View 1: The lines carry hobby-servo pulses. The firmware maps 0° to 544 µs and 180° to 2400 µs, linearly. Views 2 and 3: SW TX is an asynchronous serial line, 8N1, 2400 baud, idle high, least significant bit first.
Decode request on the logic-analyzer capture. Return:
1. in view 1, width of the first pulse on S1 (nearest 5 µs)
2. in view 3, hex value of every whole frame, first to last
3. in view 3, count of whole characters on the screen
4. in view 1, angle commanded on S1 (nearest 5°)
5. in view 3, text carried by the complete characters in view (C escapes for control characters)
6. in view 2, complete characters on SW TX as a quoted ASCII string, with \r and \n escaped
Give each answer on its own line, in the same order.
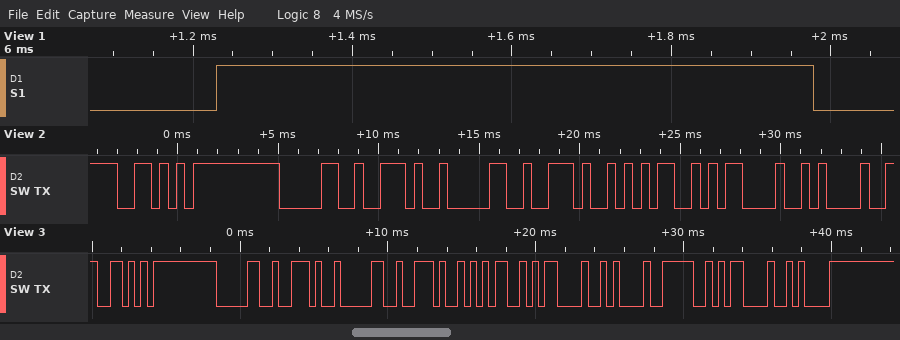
750 µs
0x56 0x30 0x2E 0x30 0x2E 0x35 0x0D 0x0A 0x3E 0x0D 0x0A
11
20°
"V0.0.5\r\n>\r\n"
"V0.0.5\r\n"
